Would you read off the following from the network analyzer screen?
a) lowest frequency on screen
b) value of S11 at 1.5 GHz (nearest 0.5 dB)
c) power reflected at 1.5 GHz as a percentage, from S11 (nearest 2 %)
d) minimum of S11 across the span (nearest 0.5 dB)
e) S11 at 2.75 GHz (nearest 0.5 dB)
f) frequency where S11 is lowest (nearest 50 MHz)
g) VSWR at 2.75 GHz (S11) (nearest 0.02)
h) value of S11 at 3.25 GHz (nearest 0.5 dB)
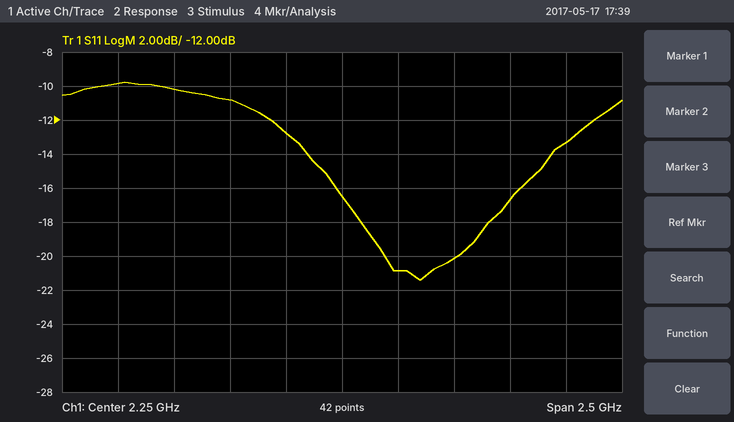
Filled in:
1 GHz
-10.0 dB
10 %
-21.5 dB
-20.0 dB
2.60 GHz
1.22
-13.5 dB
